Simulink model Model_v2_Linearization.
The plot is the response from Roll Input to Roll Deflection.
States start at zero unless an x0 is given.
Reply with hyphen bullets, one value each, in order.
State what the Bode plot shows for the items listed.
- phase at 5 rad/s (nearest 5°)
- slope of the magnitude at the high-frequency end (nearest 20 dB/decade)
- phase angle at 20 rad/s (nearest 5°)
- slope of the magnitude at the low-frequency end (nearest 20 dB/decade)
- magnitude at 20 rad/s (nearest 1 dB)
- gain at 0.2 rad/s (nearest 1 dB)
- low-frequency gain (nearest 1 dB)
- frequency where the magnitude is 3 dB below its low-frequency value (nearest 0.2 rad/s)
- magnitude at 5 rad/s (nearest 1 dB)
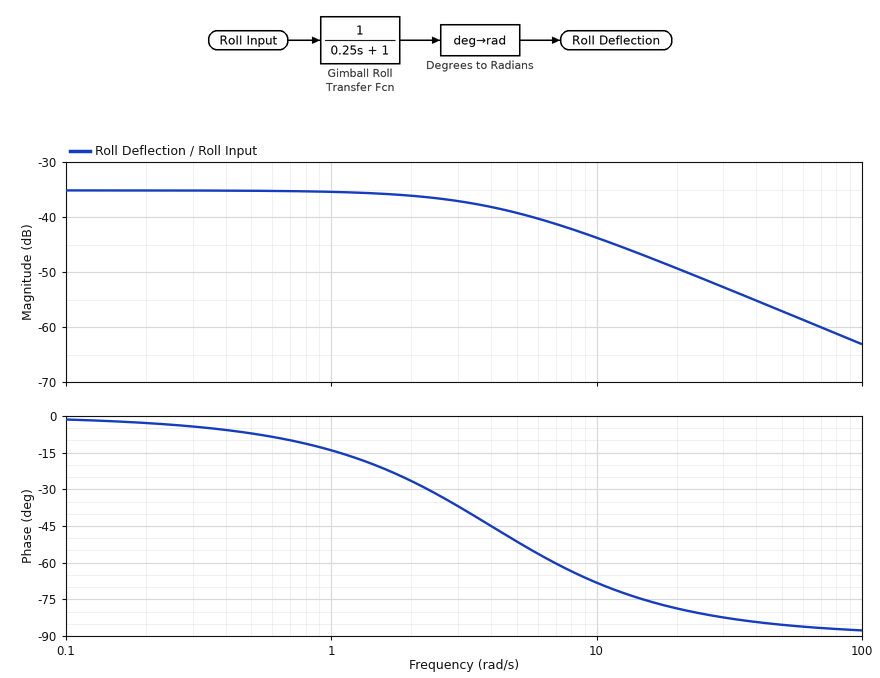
- -50°
- -20 dB/decade
- -80°
- 0 dB/decade
- -49 dB
- -35 dB
- -35 dB
- 4.0 rad/s
- -39 dB
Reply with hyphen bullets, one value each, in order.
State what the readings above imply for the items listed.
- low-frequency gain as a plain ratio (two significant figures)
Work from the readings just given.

- 0.018
